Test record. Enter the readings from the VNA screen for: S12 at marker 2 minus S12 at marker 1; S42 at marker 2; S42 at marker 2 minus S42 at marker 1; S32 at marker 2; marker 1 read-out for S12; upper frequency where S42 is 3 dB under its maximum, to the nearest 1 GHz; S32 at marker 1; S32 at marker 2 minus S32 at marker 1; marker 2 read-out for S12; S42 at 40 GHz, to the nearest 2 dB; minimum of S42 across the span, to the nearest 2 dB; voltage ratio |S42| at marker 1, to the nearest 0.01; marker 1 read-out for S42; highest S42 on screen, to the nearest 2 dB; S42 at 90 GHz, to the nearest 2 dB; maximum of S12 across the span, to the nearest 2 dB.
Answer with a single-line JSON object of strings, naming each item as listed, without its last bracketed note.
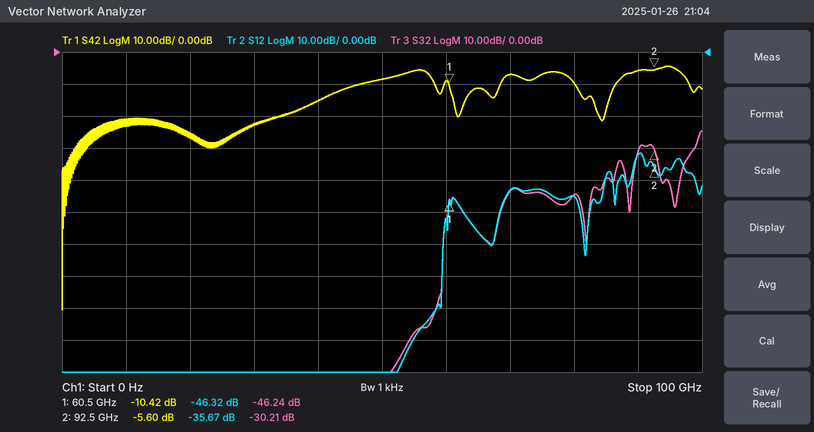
{"S12 at marker 2 minus S12 at marker 1": "10.65 dB", "S42 at marker 2": "-5.60 dB", "S42 at marker 2 minus S42 at marker 1": "4.82 dB", "S32 at marker 2": "-30.21 dB", "marker 1 read-out for S12": "-46.32 dB", "upper frequency where S42 is 3 dB under its maximum, to the nearest 1 GHz": "97 GHz", "S32 at marker 1": "-46.24 dB", "S32 at marker 2 minus S32 at marker 1": "16.03 dB", "marker 2 read-out for S12": "-35.67 dB", "S42 at 40 GHz, to the nearest 2 dB": "-16 dB", "minimum of S42 across the span, to the nearest 2 dB": "-80 dB", "voltage ratio |S42| at marker 1, to the nearest 0.01": "0.30", "marker 1 read-out for S42": "-10.42 dB", "highest S42 on screen, to the nearest 2 dB": "-4 dB", "S42 at 90 GHz, to the nearest 2 dB": "-6 dB", "maximum of S12 across the span, to the nearest 2 dB": "-32 dB"}
